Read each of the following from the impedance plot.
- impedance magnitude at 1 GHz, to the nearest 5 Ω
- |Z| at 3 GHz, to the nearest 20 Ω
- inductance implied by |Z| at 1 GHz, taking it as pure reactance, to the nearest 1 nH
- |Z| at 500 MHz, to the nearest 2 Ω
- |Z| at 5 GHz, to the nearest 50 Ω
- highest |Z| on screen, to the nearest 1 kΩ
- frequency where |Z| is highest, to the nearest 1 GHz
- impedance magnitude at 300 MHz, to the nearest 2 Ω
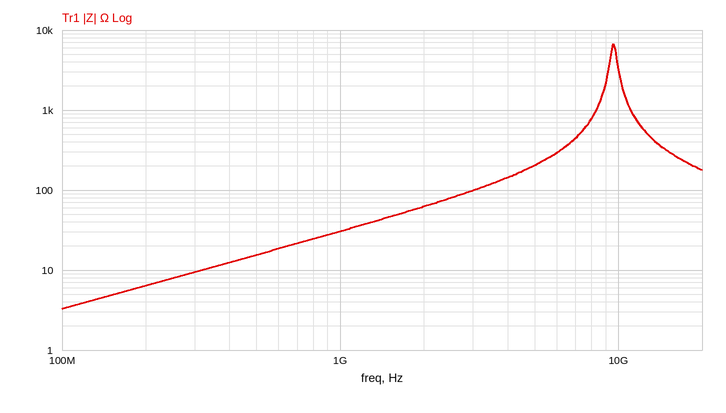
30 Ω
100 Ω
5 nH
16 Ω
200 Ω
7 kΩ
10 GHz
10 Ω
